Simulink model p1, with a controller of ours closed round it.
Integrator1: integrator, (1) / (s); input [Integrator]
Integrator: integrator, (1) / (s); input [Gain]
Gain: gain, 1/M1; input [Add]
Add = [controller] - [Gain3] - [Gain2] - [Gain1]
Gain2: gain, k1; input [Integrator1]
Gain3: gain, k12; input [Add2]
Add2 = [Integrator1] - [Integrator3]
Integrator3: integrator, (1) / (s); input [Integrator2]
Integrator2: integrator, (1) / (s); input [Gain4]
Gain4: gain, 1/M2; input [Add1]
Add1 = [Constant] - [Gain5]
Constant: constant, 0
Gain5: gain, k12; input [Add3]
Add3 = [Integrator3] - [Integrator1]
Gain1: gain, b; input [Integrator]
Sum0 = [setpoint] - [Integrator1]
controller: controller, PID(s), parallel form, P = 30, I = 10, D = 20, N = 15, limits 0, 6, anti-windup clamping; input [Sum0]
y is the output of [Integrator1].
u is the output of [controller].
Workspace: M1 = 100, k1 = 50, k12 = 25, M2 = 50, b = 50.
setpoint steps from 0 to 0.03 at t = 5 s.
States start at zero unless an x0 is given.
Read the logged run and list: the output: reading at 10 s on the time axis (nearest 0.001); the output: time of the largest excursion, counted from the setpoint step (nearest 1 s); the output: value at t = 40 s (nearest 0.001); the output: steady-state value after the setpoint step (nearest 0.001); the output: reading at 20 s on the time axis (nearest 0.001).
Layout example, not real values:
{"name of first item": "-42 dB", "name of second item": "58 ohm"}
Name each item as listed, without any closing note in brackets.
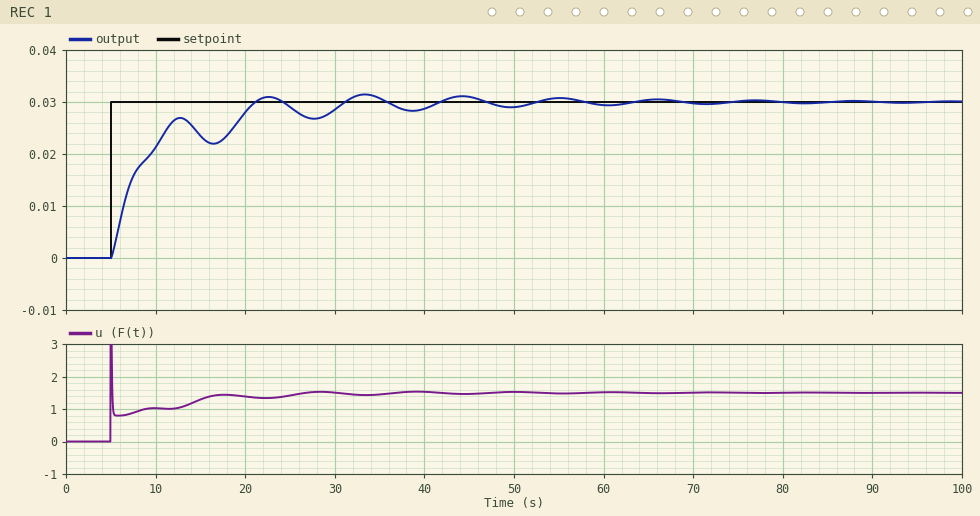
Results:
{"the output: reading at 10 s on the time axis": "0.021", "the output: time of the largest excursion, counted from the setpoint step": "28 s", "the output: value at t = 40 s": "0.029", "the output: steady-state value after the setpoint step": "0.030", "the output: reading at 20 s on the time axis": "0.028"}
